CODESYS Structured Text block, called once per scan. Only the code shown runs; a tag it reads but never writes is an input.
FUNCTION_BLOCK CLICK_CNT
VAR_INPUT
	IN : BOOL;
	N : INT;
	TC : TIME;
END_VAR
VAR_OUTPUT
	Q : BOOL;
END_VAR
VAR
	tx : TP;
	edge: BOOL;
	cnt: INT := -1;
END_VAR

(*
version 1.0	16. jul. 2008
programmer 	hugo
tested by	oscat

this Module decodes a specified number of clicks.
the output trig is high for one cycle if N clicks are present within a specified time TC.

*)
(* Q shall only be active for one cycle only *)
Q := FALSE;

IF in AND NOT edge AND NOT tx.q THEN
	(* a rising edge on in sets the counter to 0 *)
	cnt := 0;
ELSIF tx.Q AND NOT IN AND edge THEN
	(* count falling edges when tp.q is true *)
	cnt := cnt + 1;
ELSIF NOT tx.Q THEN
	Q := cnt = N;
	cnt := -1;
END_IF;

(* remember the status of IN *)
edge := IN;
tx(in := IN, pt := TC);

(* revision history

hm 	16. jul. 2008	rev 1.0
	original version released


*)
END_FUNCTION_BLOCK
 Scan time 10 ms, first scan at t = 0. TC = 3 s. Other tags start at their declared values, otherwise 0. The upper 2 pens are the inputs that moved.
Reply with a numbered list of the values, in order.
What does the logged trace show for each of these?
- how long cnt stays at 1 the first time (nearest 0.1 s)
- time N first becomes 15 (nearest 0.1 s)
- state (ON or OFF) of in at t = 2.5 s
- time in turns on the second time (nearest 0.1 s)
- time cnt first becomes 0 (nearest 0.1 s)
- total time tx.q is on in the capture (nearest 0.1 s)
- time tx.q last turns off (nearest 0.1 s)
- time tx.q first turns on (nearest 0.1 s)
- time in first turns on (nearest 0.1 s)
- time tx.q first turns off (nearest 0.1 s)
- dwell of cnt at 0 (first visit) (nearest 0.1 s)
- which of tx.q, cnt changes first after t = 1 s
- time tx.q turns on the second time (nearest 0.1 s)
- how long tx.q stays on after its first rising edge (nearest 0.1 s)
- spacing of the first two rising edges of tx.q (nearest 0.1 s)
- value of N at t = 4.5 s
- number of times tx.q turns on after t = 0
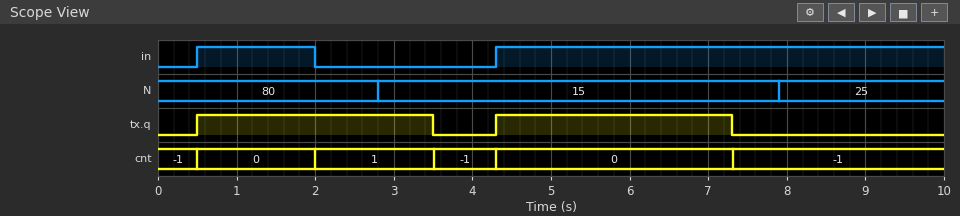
1. 1.5 s
2. 2.8 s
3. OFF
4. 4.3 s
5. 0.5 s
6. 6.0 s
7. 7.3 s
8. 0.5 s
9. 0.5 s
10. 3.5 s
11. 1.5 s
12. cnt
13. 4.3 s
14. 3.0 s
15. 3.8 s
16. 15
17. 2
